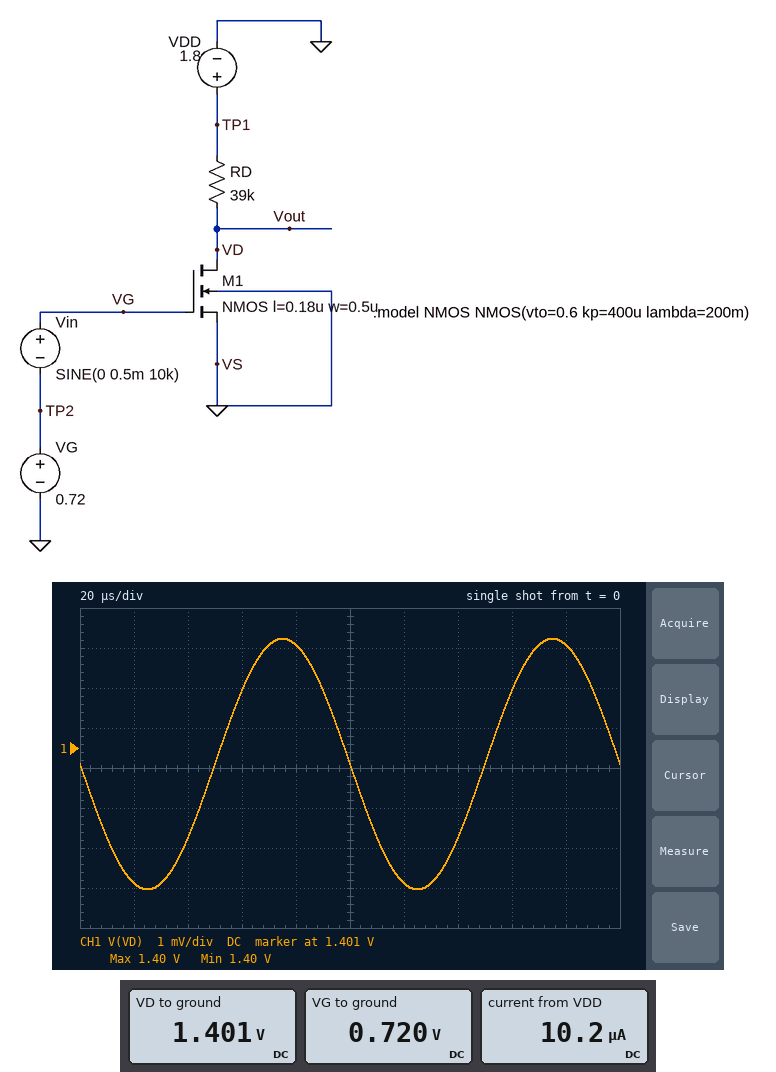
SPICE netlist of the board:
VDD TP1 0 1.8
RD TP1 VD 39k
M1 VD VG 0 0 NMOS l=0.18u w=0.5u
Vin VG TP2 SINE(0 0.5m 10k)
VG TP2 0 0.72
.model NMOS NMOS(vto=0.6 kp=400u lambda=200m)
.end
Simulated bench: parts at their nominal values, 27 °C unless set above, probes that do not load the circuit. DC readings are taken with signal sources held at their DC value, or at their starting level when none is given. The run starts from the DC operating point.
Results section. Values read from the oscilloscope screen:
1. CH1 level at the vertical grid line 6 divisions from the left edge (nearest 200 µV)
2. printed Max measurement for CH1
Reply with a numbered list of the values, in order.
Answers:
1. 1.3976 V
2. 1.40 V
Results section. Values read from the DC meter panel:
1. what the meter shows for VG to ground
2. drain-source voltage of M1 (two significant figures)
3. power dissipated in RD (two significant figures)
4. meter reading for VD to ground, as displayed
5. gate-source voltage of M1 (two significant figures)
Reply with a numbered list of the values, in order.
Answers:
1. 0.720 V
2. 1.4 V
3. 4.1 µW
4. 1.401 V
5. 720 mV
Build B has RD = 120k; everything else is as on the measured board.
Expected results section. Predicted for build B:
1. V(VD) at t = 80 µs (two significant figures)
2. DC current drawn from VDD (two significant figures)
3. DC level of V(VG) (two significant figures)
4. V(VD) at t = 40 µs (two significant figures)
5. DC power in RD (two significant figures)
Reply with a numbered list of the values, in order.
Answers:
1. 710 mV
2. 9.1 µA
3. 720 mV
4. 700 mV
5. 10 µW
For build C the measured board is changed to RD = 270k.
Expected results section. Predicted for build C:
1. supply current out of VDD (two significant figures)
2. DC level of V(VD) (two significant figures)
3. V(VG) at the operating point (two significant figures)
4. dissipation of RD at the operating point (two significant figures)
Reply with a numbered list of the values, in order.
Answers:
1. 6.4 µA
2. 65 mV
3. 720 mV
4. 11 µW
